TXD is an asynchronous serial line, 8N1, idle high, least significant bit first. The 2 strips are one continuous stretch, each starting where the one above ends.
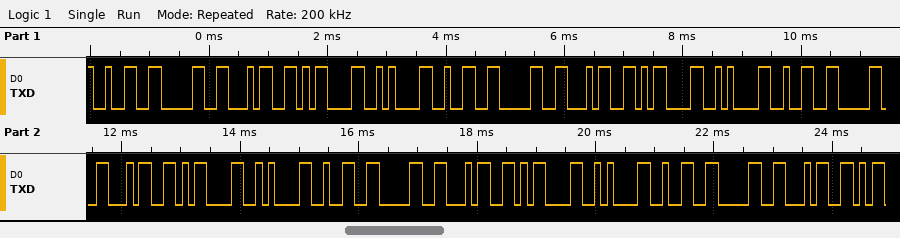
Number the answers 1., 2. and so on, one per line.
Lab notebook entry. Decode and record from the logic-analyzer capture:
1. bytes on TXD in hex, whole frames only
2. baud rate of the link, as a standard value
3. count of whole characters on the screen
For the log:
1. 32 30 34 0D 0A 32 30 34 0D 0A 32 30 34 0D 0A 32 30 34 0D 0A 32 30 34
2. 9600 baud
3. 23
